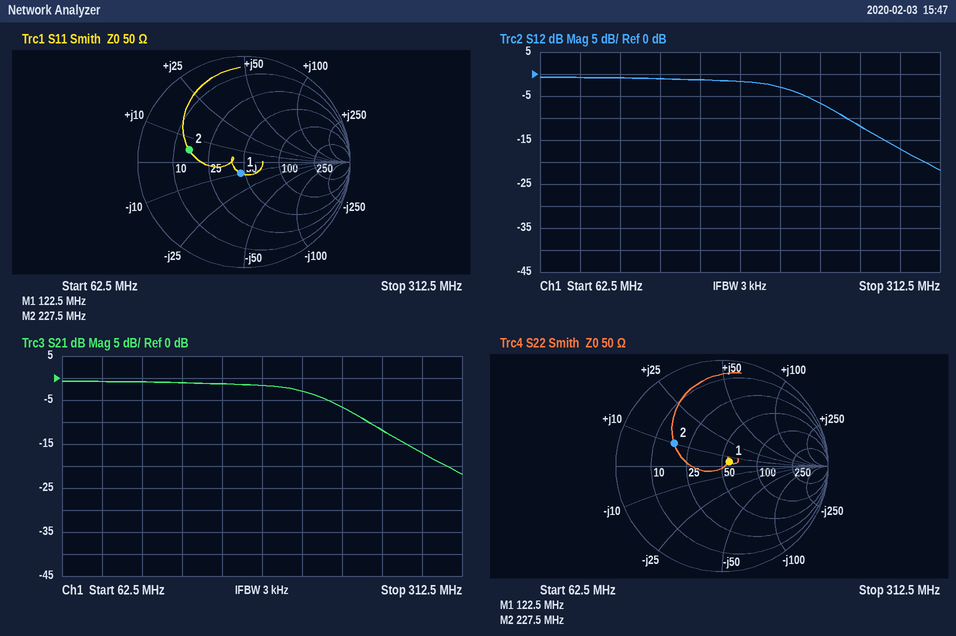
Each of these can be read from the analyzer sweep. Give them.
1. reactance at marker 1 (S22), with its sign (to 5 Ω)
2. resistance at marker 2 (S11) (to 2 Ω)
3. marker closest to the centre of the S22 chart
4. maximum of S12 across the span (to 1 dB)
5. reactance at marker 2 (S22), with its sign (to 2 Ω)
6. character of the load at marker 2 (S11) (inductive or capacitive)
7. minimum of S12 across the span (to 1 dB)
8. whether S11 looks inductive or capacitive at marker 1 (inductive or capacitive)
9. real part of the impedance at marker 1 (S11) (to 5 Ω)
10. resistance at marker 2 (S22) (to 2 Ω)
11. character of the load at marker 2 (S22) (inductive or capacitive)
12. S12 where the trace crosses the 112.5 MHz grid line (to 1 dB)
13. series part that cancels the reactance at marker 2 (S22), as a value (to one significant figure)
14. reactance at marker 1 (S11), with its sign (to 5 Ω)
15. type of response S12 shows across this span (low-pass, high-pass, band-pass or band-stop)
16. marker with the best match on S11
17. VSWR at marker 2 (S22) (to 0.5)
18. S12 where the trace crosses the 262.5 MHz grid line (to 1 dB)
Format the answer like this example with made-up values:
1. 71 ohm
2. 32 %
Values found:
1. +5 Ω
2. 16 Ω
3. marker 1
4. -1 dB
5. +10 Ω
6. inductive
7. -22 dB
8. capacitive
9. 45 Ω
10. 18 Ω
11. inductive
12. -1 dB
13. 70 pF
14. -10 Ω
15. low-pass
16. marker 1
17. 3.0
18. -12 dB
